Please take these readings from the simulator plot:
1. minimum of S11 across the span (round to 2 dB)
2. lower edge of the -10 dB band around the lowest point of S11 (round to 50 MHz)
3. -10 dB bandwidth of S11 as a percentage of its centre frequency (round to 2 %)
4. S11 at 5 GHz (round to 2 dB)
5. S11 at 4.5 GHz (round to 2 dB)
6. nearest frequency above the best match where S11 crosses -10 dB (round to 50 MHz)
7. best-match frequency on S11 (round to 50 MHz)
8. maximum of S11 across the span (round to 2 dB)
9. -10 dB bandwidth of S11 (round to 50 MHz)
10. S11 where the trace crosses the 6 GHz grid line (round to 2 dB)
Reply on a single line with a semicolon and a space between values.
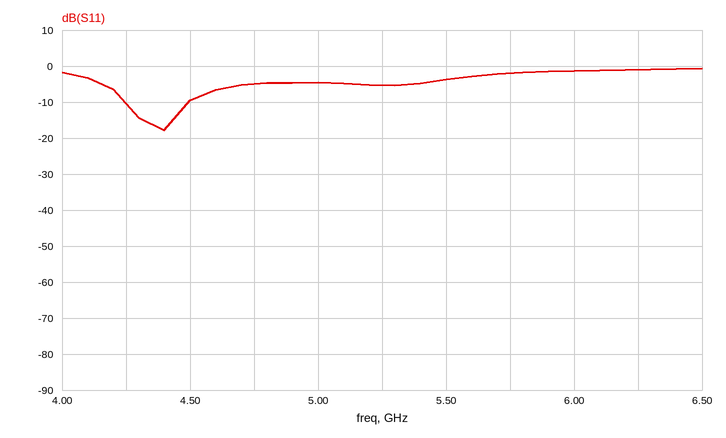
-18 dB; 4.25 GHz; 6 %; -4 dB; -10 dB; 4.50 GHz; 4.40 GHz; 0 dB; 250 MHz; -2 dB
